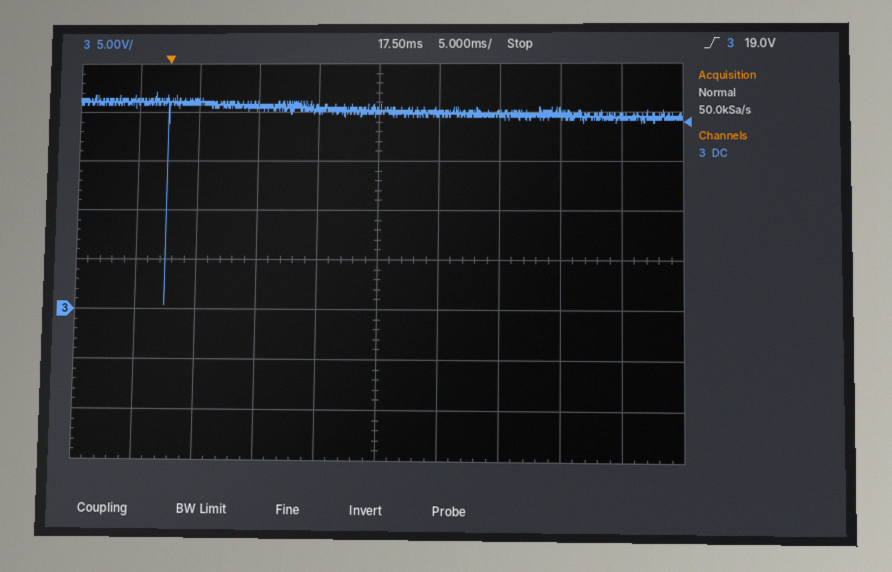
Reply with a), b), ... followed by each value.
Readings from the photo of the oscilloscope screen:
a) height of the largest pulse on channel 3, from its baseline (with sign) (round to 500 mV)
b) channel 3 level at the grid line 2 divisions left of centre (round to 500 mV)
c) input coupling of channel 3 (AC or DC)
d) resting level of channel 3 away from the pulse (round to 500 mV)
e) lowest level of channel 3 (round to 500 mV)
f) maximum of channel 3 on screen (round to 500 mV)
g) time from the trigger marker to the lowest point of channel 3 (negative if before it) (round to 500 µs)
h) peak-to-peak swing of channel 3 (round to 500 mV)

a) -19.5 V
b) 20.5 V
c) DC
d) 20.0 V
e) 500 mV
f) 22.0 V
g) 0.0 ms
h) 21.5 V
